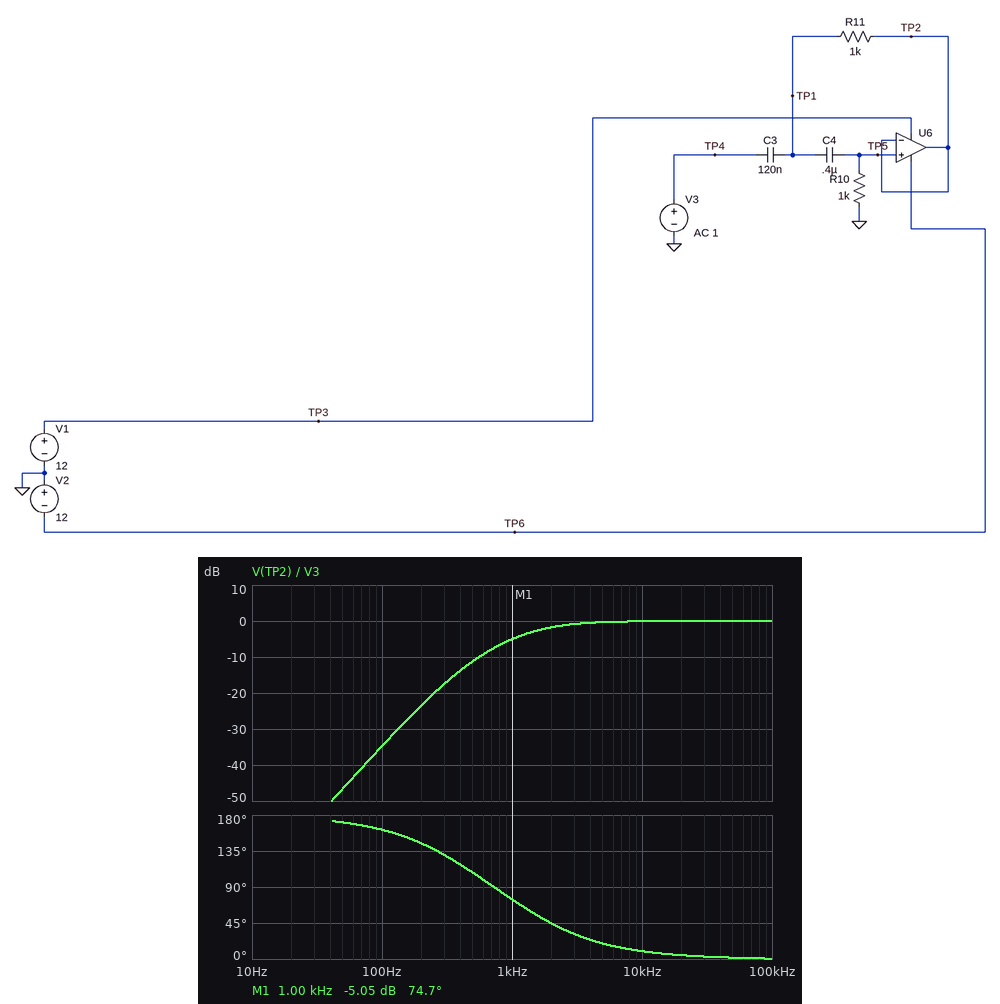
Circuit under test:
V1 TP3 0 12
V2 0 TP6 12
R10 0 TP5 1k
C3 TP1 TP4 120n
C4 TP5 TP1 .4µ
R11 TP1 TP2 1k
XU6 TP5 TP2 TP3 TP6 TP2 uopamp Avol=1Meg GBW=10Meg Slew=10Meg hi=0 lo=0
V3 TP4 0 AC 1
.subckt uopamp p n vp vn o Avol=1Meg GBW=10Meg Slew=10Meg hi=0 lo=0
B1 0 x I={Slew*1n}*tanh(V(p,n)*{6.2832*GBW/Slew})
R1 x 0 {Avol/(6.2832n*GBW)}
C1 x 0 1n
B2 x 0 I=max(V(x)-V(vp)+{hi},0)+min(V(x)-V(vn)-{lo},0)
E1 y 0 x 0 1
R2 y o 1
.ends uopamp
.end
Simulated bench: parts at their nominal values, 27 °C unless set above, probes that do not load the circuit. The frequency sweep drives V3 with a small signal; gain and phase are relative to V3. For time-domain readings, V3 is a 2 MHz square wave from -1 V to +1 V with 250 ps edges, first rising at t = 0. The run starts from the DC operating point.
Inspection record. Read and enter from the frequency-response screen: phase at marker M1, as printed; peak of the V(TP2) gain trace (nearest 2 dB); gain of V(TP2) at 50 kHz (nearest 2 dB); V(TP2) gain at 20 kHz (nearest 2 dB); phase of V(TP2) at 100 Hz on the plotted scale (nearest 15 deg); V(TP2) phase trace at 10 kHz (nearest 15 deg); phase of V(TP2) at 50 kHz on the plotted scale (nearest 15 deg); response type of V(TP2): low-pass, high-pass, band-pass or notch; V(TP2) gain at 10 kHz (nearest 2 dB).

74.7 deg
0 dB
0 dB
0 dB
165 deg
15 deg
0 deg
high-pass
0 dB
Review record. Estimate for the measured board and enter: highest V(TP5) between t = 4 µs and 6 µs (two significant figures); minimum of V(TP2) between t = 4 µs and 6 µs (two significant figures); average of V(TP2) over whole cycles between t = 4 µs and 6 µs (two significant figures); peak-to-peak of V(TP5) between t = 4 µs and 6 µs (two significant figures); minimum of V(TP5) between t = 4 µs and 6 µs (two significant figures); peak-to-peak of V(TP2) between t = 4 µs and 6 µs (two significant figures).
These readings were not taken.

2.0 V
-60 mV
950 mV
2.0 V
-65 mV
2.0 V
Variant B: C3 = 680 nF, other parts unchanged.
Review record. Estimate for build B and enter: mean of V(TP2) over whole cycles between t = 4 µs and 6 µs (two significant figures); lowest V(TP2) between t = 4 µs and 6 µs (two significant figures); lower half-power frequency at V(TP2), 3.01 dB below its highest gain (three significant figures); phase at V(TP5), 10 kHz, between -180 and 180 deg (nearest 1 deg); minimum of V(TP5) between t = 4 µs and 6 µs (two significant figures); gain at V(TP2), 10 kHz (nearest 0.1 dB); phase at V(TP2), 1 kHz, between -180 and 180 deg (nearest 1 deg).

980 mV
-20 mV
498 Hz
4 deg
-24 mV
0 dB
35 deg
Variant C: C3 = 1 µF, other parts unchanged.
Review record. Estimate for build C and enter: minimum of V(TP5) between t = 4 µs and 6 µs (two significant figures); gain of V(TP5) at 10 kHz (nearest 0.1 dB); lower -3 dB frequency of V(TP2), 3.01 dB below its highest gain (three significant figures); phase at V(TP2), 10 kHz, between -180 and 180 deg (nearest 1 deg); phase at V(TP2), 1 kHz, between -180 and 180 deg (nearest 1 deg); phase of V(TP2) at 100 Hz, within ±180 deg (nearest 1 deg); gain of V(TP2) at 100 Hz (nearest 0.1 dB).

-21 mV
0 dB
451 Hz
3 deg
31 deg
134 deg
-17.7 dB
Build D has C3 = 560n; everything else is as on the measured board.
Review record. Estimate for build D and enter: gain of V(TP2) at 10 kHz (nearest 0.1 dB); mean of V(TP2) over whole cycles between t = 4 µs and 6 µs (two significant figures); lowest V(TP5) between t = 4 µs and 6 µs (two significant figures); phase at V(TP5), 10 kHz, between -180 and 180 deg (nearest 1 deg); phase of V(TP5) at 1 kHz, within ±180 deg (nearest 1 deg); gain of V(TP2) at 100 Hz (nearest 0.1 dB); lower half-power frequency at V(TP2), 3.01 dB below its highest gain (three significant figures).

0 dB
980 mV
-26 mV
4 deg
38 deg
-21.8 dB
533 Hz
